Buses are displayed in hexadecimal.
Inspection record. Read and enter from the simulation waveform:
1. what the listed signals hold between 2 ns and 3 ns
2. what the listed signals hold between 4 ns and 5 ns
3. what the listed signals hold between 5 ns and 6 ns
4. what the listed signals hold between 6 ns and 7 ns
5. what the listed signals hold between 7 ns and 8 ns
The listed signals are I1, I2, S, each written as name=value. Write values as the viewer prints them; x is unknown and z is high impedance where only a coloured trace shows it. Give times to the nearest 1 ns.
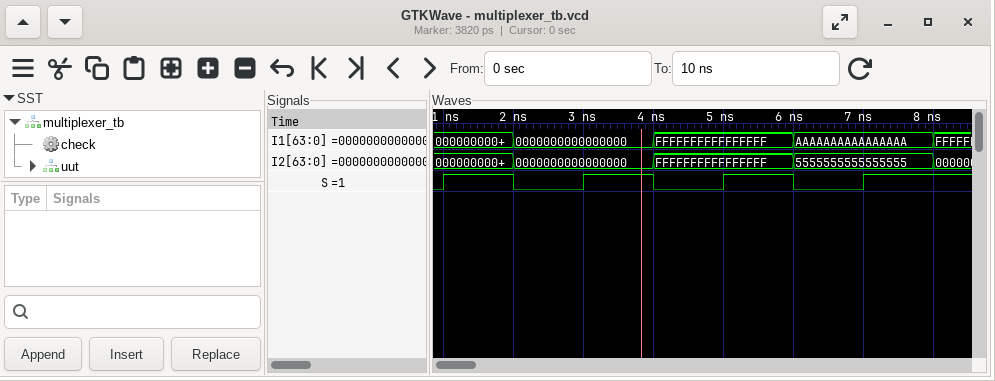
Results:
I1=0000000000000000, I2=0000000000000000, S=0
I1=FFFFFFFFFFFFFFFF, I2=FFFFFFFFFFFFFFFF, S=0
I1=FFFFFFFFFFFFFFFF, I2=FFFFFFFFFFFFFFFF, S=1
I1=AAAAAAAAAAAAAAAA, I2=5555555555555555, S=0
I1=AAAAAAAAAAAAAAAA, I2=5555555555555555, S=1
